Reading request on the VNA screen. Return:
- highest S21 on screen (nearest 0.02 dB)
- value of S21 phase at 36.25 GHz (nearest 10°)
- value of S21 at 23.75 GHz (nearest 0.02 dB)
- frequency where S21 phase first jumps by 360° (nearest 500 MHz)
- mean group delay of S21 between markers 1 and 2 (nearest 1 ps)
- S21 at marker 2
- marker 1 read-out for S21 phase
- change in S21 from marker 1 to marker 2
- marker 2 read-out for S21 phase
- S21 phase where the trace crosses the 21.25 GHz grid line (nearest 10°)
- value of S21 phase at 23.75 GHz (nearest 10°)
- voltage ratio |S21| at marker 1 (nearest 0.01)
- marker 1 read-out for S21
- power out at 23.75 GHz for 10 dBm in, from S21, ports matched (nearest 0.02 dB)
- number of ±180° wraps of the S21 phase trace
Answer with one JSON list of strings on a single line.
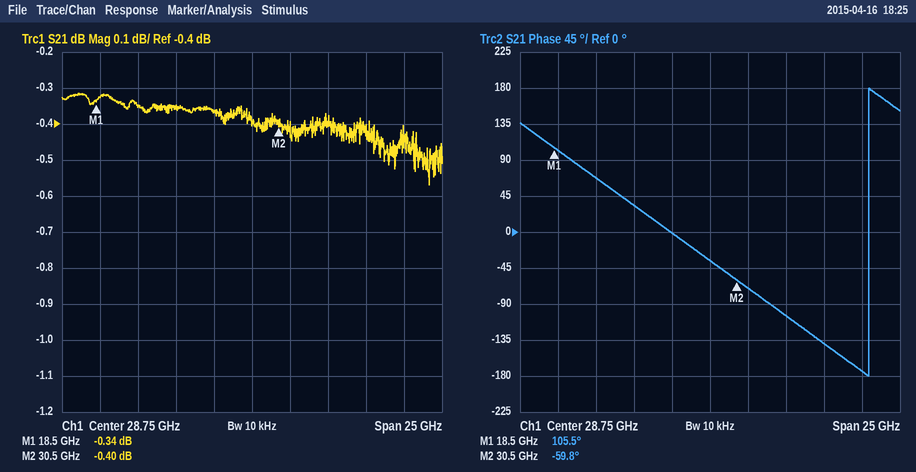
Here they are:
["-0.32 dB", "-140°", "-0.36 dB", "39.0 GHz", "38 ps", "-0.40 dB", "105.5°", "-0.06 dB", "-59.8°", "70°", "30°", "0.96", "-0.34 dB", "9.64 dBm", "1"]
